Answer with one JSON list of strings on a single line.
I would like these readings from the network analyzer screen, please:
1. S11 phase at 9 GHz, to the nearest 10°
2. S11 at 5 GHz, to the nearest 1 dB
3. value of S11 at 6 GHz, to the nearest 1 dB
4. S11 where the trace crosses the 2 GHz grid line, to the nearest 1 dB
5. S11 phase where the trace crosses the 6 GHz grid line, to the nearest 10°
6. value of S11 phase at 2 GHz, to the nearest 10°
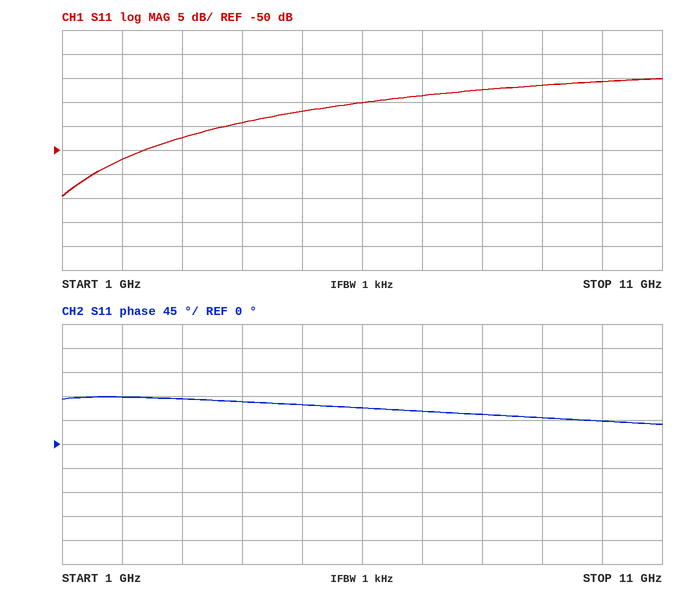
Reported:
["50°", "-42 dB", "-40 dB", "-52 dB", "70°", "90°"]
